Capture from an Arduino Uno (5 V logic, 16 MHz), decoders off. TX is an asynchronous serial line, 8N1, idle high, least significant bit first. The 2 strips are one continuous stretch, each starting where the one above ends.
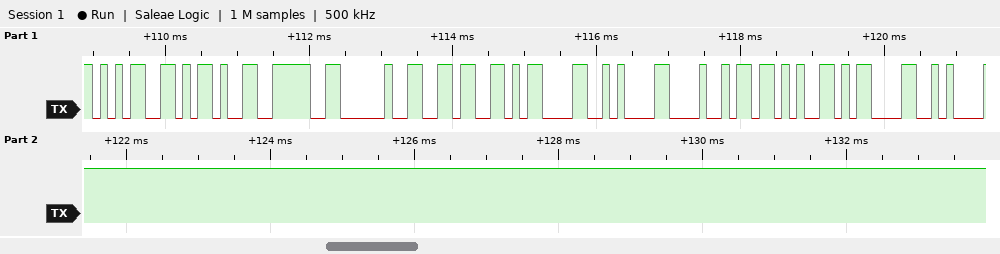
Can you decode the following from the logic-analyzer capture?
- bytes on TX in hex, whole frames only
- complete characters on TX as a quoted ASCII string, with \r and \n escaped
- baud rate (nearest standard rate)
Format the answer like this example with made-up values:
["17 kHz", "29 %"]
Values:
["35 2D 3E 20 36 0D 0A 48 2B 0D 0A", "\"5-> 6\\r\\nH+\\r\\n\"", "9600 baud"]
